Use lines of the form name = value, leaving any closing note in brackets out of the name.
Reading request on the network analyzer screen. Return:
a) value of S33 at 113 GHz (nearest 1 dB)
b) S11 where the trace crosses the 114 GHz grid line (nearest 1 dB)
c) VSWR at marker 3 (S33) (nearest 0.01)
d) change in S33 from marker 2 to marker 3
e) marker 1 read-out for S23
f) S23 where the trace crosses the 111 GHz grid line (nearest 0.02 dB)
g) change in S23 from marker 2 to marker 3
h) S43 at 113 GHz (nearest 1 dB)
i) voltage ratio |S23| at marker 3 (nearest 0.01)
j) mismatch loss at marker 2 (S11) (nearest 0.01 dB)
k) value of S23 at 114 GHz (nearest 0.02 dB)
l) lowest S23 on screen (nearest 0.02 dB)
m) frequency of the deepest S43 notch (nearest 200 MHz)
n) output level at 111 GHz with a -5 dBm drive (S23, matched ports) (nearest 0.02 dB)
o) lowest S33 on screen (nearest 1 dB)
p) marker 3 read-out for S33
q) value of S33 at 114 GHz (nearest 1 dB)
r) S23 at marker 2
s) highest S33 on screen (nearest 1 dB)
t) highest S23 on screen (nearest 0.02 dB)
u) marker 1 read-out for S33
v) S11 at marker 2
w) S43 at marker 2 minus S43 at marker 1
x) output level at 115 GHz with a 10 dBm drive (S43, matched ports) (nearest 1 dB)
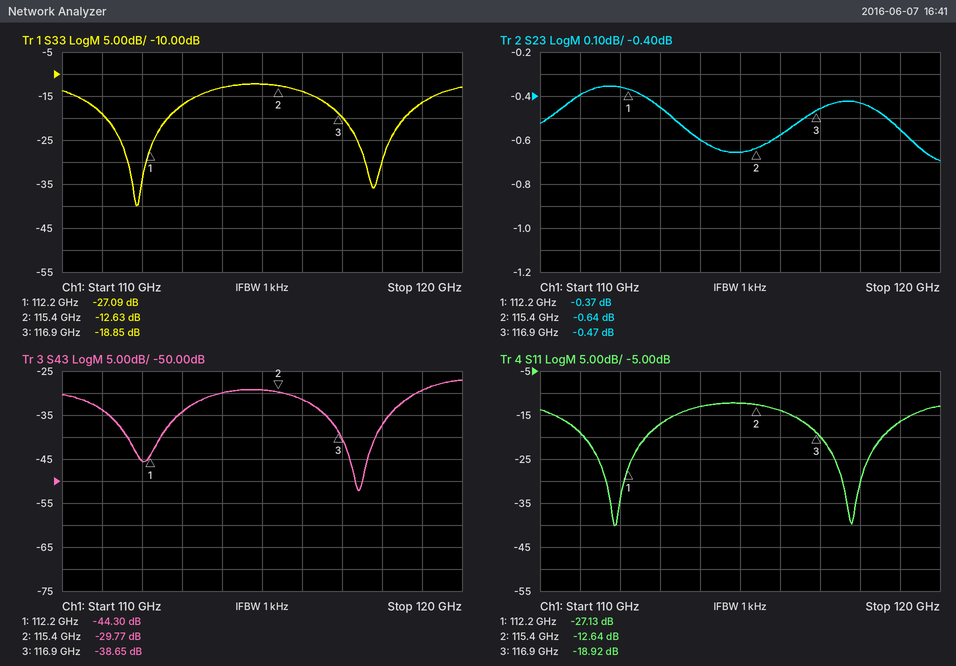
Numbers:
value of S33 at 113 GHz = -17 dB
S11 where the trace crosses the 114 GHz grid line = -13 dB
VSWR at marker 3 (S33) = 1.26
change in S33 from marker 2 to marker 3 = -6.22 dB
marker 1 read-out for S23 = -0.37 dB
S23 where the trace crosses the 111 GHz grid line = -0.40 dB
change in S23 from marker 2 to marker 3 = 0.17 dB
S43 at 113 GHz = -34 dB
voltage ratio |S23| at marker 3 = 0.95
mismatch loss at marker 2 (S11) = 0.24 dB
value of S23 at 114 GHz = -0.60 dB
lowest S23 on screen = -0.70 dB
frequency of the deepest S43 notch = 117.4 GHz
output level at 111 GHz with a -5 dBm drive (S23, matched ports) = -5.40 dBm
lowest S33 on screen = -40 dB
marker 3 read-out for S33 = -18.85 dB
value of S33 at 114 GHz = -13 dB
S23 at marker 2 = -0.64 dB
highest S33 on screen = -12 dB
highest S23 on screen = -0.36 dB
marker 1 read-out for S33 = -27.09 dB
S11 at marker 2 = -12.64 dB
S43 at marker 2 minus S43 at marker 1 = 14.53 dB
output level at 115 GHz with a 10 dBm drive (S43, matched ports) = -19 dBm
